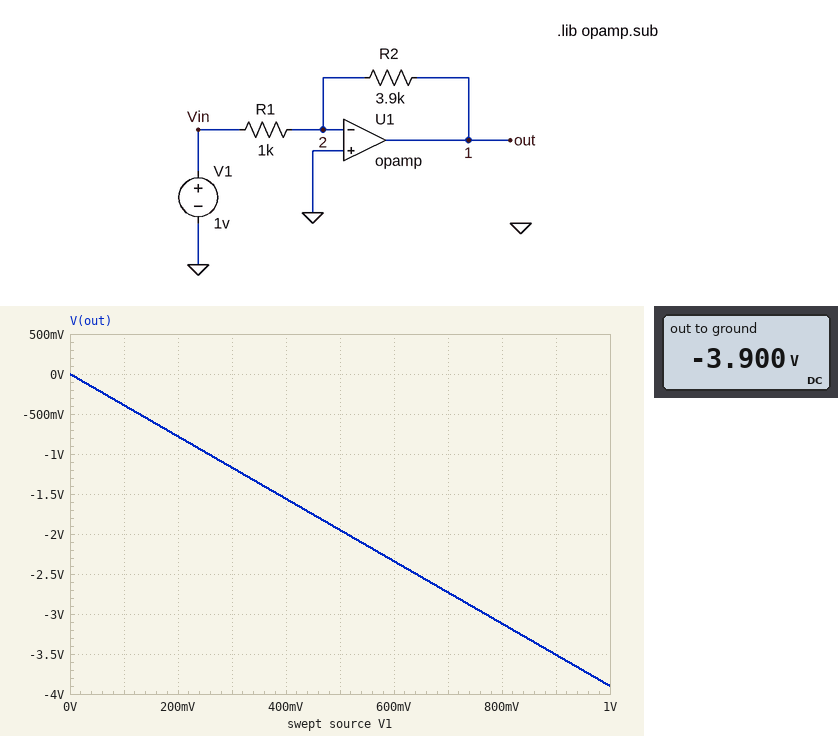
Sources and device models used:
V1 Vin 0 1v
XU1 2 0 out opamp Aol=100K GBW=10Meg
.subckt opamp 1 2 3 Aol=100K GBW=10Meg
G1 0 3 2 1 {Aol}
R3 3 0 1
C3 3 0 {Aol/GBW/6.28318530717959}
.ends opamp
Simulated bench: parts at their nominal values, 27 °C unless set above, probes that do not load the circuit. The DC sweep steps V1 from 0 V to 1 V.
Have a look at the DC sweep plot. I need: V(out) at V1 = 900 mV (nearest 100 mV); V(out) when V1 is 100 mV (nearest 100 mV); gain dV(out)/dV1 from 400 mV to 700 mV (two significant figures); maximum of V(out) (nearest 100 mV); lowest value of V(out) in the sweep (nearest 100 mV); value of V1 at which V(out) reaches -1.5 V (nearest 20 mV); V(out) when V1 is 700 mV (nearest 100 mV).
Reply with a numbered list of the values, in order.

1. -3.5 V
2. -400 mV
3. -3.9 V/V
4. 0 V
5. -3.9 V
6. 380 mV
7. -2.7 V
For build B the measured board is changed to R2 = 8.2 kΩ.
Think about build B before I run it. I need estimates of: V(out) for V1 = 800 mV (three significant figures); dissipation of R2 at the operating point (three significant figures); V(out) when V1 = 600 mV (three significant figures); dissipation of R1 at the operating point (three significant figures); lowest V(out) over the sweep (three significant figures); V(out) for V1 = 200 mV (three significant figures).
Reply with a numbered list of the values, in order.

1. -6.56 V
2. 8.20 mW
3. -4.92 V
4. 1.00 mW
5. -8.20 V
6. -1.64 V
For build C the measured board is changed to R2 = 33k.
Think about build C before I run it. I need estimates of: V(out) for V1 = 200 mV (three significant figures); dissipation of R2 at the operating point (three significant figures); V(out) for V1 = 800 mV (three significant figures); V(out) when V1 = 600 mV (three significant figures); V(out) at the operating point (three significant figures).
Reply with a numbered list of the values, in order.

1. -6.60 V
2. 33.0 mW
3. -26.4 V
4. -19.8 V
5. -33.0 V
